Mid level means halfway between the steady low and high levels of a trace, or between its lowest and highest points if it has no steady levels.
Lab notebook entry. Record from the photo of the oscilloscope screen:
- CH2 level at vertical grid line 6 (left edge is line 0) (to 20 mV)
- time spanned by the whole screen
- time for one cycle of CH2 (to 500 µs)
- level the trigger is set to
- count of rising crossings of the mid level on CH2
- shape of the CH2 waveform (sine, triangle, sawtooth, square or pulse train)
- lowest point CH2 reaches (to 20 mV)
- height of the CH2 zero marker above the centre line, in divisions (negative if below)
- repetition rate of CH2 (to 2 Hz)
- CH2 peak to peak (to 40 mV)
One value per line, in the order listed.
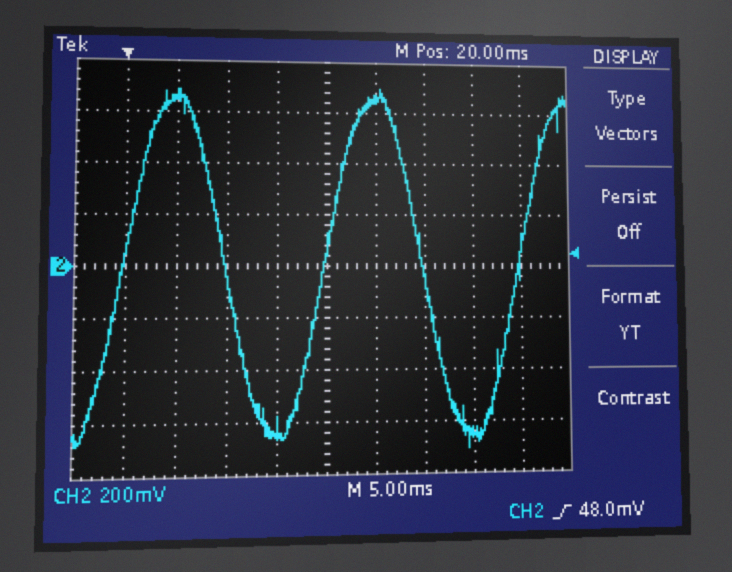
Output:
660 mV
50 ms
20.0 ms
48.0 mV
3
sine
-700 mV
0.0 div
50 Hz
1.40 V
